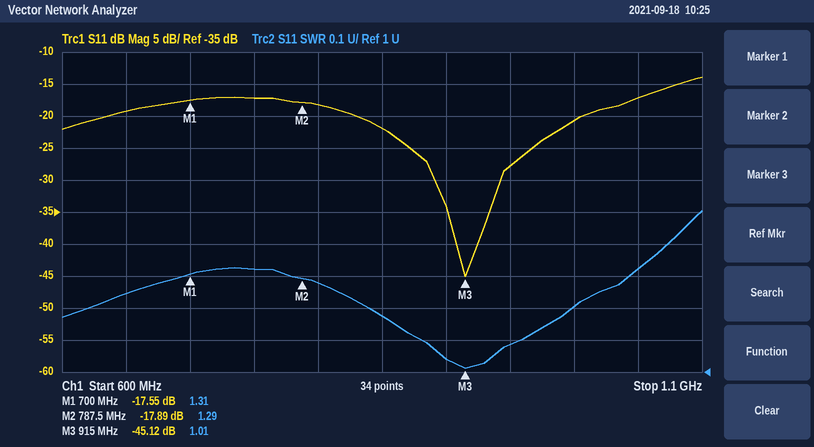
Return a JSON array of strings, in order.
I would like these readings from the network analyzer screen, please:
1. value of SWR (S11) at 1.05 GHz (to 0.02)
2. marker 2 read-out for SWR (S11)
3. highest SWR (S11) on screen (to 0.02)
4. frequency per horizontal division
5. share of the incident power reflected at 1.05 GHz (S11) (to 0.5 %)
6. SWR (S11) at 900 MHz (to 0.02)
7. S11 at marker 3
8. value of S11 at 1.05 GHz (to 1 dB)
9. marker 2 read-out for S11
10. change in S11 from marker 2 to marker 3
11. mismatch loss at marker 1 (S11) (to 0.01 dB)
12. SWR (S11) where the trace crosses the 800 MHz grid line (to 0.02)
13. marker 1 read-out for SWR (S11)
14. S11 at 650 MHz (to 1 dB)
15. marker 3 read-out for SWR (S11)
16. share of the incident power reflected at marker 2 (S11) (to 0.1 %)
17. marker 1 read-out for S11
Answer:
["1.32", "1.29", "1.50", "50 MHz", "2.0 %", "1.04", "-45.12 dB", "-17 dB", "-17.89 dB", "-27.23 dB", "0.08 dB", "1.28", "1.31", "-19 dB", "1.01", "1.6 %", "-17.55 dB"]
